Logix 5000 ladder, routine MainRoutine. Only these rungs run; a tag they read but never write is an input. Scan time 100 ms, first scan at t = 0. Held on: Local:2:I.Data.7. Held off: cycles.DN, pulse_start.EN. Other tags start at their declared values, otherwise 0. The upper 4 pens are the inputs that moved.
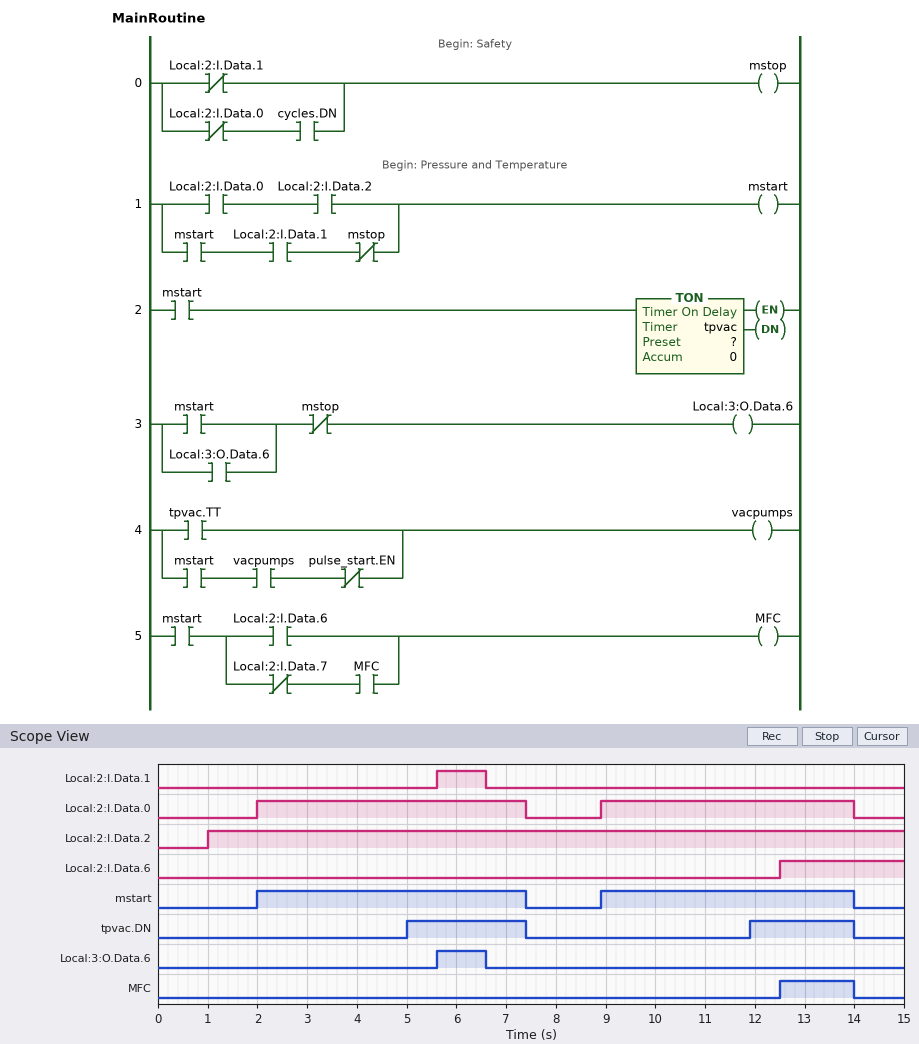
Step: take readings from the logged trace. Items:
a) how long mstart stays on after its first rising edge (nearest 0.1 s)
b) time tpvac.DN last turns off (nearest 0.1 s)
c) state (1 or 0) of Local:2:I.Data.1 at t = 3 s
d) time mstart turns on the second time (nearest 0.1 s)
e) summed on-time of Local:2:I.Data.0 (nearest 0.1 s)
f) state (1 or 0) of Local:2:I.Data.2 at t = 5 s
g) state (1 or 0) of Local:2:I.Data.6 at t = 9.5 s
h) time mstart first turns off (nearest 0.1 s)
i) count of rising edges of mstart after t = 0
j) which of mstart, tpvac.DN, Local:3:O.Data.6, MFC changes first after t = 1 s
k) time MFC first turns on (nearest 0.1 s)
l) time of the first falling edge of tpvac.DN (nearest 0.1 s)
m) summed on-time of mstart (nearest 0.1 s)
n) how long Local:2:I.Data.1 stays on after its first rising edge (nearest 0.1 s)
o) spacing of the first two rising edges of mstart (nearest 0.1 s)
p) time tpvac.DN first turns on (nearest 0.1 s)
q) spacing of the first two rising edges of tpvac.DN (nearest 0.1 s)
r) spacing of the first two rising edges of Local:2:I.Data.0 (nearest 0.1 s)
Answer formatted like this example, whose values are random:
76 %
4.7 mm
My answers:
5.4 s
14.0 s
0
8.9 s
10.5 s
1
0
7.4 s
2
mstart
12.5 s
7.4 s
10.5 s
1.0 s
6.9 s
5.0 s
6.9 s
6.9 s
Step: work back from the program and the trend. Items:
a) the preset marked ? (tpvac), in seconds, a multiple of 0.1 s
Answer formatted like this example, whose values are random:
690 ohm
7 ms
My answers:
3.0 s
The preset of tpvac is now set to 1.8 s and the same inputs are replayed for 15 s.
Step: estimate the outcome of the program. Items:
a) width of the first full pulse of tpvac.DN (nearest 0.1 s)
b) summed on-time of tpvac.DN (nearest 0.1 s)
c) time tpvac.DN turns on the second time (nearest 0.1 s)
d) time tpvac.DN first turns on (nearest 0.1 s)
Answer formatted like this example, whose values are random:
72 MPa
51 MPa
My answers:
3.6 s
6.9 s
10.7 s
3.8 s
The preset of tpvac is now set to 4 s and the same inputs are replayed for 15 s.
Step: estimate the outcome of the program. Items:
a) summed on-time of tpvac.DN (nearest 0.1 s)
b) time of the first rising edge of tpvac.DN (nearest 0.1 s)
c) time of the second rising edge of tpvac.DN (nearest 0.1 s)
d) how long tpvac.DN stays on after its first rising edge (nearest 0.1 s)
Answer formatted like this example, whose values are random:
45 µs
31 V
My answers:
2.5 s
6.0 s
12.9 s
1.4 s
